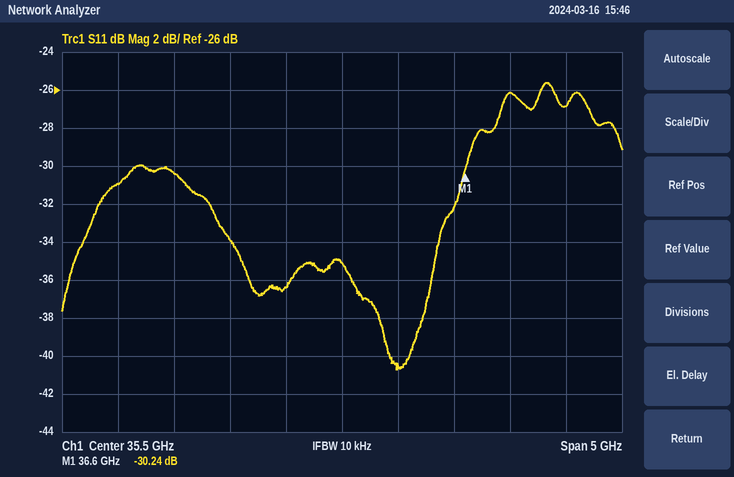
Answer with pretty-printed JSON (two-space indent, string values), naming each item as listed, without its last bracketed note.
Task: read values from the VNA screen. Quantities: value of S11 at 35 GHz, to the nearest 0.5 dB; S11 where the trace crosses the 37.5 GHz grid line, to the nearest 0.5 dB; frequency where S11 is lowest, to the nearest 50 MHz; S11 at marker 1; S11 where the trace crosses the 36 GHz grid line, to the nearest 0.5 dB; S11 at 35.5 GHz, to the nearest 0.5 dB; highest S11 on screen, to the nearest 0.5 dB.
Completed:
{
  "value of S11 at 35 GHz, to the nearest 0.5 dB": "-36.5 dB",
  "S11 where the trace crosses the 37.5 GHz grid line, to the nearest 0.5 dB": "-27.0 dB",
  "frequency where S11 is lowest, to the nearest 50 MHz": "36.00 GHz",
  "S11 at marker 1": "-30.24 dB",
  "S11 where the trace crosses the 36 GHz grid line, to the nearest 0.5 dB": "-40.5 dB",
  "S11 at 35.5 GHz, to the nearest 0.5 dB": "-35.0 dB",
  "highest S11 on screen, to the nearest 0.5 dB": "-25.5 dB"
}
